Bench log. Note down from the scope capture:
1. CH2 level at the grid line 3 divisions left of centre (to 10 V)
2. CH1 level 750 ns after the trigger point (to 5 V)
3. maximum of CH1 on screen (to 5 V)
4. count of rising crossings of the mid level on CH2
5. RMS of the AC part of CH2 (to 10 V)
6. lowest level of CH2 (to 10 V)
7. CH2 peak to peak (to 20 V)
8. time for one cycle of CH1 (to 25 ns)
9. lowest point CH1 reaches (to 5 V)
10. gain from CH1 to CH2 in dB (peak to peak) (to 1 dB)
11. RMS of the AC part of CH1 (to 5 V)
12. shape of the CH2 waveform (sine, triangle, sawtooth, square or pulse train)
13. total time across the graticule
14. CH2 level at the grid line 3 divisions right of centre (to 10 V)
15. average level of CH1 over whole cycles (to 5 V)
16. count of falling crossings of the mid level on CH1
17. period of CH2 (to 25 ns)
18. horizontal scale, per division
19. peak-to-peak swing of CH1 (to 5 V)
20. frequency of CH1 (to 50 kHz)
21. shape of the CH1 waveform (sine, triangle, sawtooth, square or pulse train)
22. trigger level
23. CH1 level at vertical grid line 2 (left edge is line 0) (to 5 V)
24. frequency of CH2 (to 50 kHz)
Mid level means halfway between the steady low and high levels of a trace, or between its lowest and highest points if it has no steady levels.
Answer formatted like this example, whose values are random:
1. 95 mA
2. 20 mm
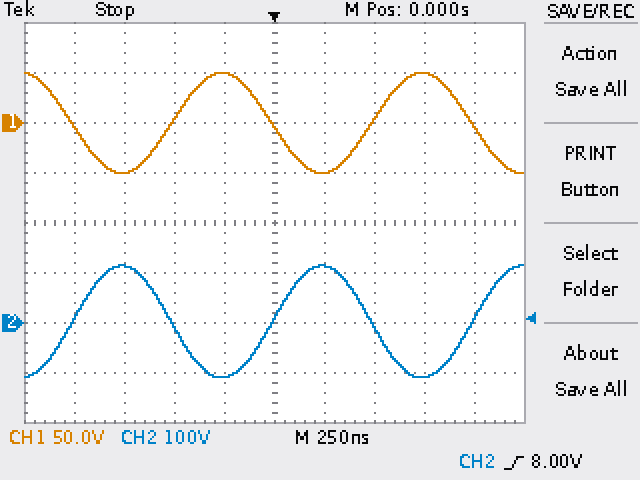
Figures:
1. 110 V
2. 50 V
3. 50 V
4. 3
5. 80 V
6. -110 V
7. 220 V
8. 1.000 µs
9. -50 V
10. 7 dB
11. 35 V
12. sine
13. 2.5 µs
14. -110 V
15. 0 V
16. 3
17. 1.000 µs
18. 250 ns
19. 100 V
20. 1.00 MHz
21. sine
22. 8.00 V
23. -50 V
24. 1.00 MHz
